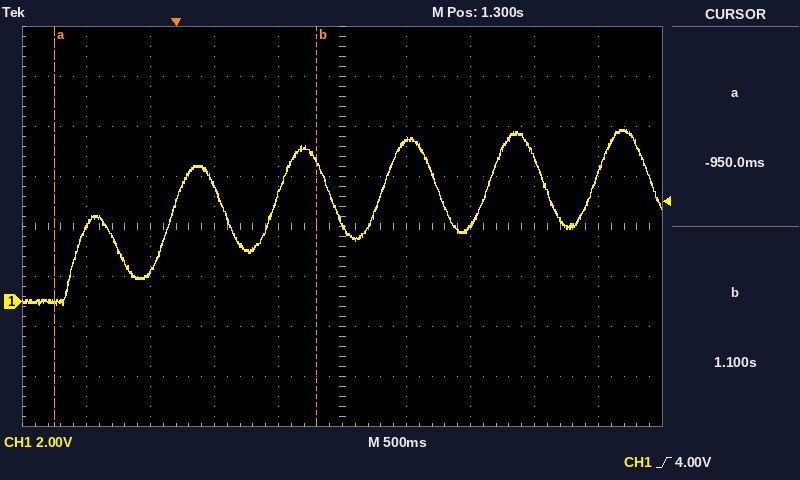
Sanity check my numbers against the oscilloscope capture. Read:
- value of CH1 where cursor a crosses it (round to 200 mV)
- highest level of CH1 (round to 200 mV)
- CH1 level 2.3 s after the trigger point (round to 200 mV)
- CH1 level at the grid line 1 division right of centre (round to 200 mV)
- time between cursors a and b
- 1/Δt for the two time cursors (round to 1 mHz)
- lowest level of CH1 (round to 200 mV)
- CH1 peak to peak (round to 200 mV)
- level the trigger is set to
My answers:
0.0 V
6.8 V
3.0 V
6.4 V
2.05 s
488 mHz
-200 mV
7.0 V
4.00 V
